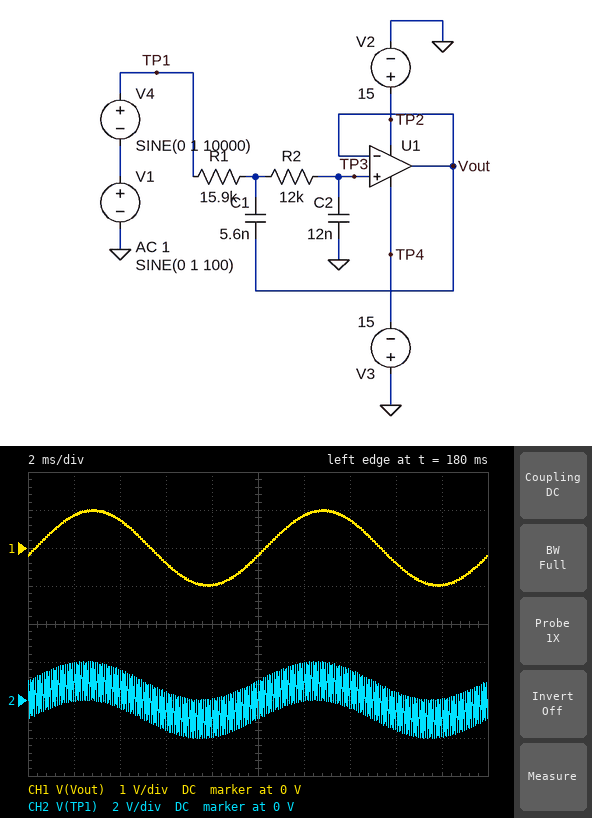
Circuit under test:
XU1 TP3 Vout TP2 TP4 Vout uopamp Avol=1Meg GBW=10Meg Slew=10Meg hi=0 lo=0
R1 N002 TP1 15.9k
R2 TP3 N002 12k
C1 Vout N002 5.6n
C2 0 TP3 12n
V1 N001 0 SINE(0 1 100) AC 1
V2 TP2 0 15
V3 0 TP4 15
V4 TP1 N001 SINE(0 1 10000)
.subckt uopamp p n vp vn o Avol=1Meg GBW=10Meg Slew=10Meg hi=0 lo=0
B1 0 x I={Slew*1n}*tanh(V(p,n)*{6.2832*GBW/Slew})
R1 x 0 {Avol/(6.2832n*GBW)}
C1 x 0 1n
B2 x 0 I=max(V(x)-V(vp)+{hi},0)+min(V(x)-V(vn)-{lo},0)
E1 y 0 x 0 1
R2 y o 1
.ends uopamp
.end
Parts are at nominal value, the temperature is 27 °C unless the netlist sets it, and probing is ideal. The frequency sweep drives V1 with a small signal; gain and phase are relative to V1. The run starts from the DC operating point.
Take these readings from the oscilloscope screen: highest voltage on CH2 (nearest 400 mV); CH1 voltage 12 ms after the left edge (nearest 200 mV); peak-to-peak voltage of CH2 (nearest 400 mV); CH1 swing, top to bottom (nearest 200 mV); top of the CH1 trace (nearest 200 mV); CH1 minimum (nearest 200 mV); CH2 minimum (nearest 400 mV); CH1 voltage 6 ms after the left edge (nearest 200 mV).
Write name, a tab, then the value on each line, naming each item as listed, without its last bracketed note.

highest voltage on CH2	2.0 V
CH1 voltage 12 ms after the left edge	800 mV
peak-to-peak voltage of CH2	4.0 V
CH1 swing, top to bottom	2.0 V
top of the CH1 trace	1.0 V
CH1 minimum	-1.0 V
CH2 minimum	-2.0 V
CH1 voltage 6 ms after the left edge	-400 mV
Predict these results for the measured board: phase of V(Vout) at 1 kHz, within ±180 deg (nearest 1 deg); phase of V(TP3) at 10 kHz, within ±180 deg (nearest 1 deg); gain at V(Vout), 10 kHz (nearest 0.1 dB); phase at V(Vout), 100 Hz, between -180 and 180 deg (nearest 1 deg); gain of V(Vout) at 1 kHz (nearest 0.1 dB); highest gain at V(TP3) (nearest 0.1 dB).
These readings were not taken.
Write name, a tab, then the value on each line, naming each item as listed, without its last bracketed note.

phase of V(Vout) at 1 kHz, within ±180 deg	-77 deg
phase of V(TP3) at 10 kHz, within ±180 deg	-157 deg
gain at V(Vout), 10 kHz	-34.6 dB
phase at V(Vout), 100 Hz, between -180 and 180 deg	-12 deg
gain of V(Vout) at 1 kHz	-6.7 dB
highest gain at V(TP3)	0 dB
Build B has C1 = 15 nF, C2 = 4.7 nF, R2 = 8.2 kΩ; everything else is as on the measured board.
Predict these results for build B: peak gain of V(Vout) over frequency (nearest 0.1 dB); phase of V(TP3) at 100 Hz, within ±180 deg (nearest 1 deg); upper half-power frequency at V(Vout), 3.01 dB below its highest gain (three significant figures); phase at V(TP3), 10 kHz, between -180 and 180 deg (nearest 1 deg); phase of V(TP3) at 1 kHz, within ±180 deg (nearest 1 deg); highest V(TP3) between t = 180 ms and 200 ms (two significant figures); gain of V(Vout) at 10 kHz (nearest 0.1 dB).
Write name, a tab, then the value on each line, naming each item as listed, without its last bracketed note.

peak gain of V(Vout) over frequency	0.4 dB
phase of V(TP3) at 100 Hz, within ±180 deg	-4 deg
upper half-power frequency at V(Vout), 3.01 dB below its highest gain	1.86 kHz
phase at V(TP3), 10 kHz, between -180 and 180 deg	-169 deg
phase of V(TP3) at 1 kHz, within ±180 deg	-48 deg
highest V(TP3) between t = 180 ms and 200 ms	1.0 V
gain of V(Vout) at 10 kHz	-31.1 dB
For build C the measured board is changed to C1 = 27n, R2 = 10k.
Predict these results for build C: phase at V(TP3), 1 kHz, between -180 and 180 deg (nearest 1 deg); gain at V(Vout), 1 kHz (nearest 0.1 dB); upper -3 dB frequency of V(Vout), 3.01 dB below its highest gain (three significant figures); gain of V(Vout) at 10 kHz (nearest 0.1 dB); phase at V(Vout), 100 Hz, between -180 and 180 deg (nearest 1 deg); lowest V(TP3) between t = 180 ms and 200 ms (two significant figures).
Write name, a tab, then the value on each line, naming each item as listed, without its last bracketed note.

phase at V(TP3), 1 kHz, between -180 and 180 deg	-118 deg
gain at V(Vout), 1 kHz	-6.9 dB
upper -3 dB frequency of V(Vout), 3.01 dB below its highest gain	722 Hz
gain of V(Vout) at 10 kHz	-46.2 dB
phase at V(Vout), 100 Hz, between -180 and 180 deg	-11 deg
lowest V(TP3) between t = 180 ms and 200 ms	-1.0 V
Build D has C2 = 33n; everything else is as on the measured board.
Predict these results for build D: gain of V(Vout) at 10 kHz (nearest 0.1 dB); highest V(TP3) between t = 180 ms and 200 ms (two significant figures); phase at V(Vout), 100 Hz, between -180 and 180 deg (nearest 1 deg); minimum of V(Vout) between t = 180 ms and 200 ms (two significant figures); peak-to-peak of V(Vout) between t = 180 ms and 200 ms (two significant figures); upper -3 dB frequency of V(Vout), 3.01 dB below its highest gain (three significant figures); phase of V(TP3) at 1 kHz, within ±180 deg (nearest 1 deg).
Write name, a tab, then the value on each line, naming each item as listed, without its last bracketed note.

gain of V(Vout) at 10 kHz	-43.5 dB
highest V(TP3) between t = 180 ms and 200 ms	880 mV
phase at V(Vout), 100 Hz, between -180 and 180 deg	-30 deg
minimum of V(Vout) between t = 180 ms and 200 ms	-880 mV
peak-to-peak of V(Vout) between t = 180 ms and 200 ms	1.8 V
upper -3 dB frequency of V(Vout), 3.01 dB below its highest gain	180 Hz
phase of V(TP3) at 1 kHz, within ±180 deg	-94 deg
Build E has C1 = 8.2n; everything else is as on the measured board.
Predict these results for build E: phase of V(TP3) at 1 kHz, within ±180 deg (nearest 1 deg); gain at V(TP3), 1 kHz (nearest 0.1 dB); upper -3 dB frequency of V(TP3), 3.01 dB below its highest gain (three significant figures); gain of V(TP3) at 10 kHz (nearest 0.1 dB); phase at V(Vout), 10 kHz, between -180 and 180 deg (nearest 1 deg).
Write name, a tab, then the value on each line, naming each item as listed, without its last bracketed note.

phase of V(TP3) at 1 kHz, within ±180 deg	-83 deg
gain at V(TP3), 1 kHz	-6.5 dB
upper -3 dB frequency of V(TP3), 3.01 dB below its highest gain	566 Hz
gain of V(TP3) at 10 kHz	-37.6 dB
phase at V(Vout), 10 kHz, between -180 and 180 deg	-164 deg
